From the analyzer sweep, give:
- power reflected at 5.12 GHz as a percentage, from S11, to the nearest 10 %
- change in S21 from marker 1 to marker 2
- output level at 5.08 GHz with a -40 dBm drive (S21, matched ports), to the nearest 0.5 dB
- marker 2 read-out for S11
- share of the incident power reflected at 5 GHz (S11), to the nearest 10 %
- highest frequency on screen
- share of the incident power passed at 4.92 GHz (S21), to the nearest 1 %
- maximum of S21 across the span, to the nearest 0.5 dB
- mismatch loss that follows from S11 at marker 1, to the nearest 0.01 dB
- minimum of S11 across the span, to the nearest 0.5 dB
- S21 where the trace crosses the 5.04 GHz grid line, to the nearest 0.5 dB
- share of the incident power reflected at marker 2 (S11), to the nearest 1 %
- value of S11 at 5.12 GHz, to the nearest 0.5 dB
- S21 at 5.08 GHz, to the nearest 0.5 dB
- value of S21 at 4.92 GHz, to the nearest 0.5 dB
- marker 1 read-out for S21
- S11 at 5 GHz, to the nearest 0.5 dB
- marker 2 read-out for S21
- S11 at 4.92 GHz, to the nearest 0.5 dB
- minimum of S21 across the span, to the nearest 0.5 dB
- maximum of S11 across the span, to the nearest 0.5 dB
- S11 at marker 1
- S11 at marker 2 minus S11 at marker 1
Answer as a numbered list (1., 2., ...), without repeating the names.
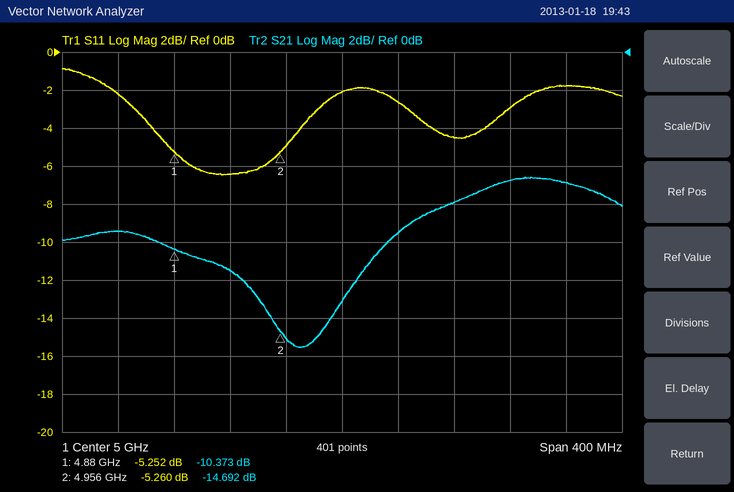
1. 50 %
2. -4.319 dB
3. -48.0 dBm
4. -5.260 dB
5. 60 %
6. 5.2 GHz
7. 7 %
8. -6.5 dB
9. 1.54 dB
10. -6.5 dB
11. -9.5 dB
12. 30 %
13. -3.0 dB
14. -8.0 dB
15. -11.5 dB
16. -10.373 dB
17. -2.0 dB
18. -14.692 dB
19. -6.5 dB
20. -15.5 dB
21. -1.0 dB
22. -5.252 dB
23. -0.008 dB
